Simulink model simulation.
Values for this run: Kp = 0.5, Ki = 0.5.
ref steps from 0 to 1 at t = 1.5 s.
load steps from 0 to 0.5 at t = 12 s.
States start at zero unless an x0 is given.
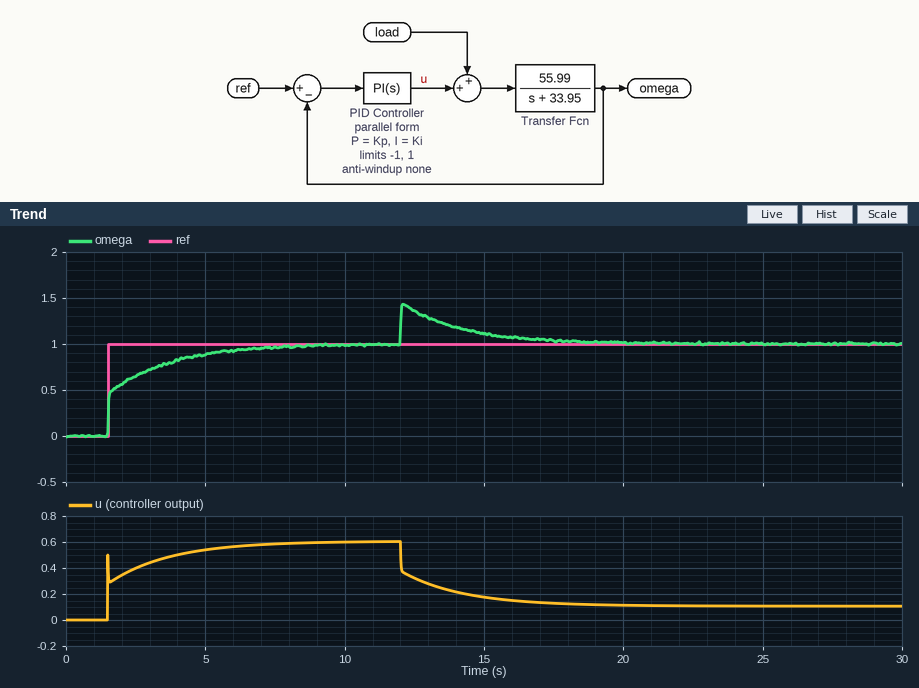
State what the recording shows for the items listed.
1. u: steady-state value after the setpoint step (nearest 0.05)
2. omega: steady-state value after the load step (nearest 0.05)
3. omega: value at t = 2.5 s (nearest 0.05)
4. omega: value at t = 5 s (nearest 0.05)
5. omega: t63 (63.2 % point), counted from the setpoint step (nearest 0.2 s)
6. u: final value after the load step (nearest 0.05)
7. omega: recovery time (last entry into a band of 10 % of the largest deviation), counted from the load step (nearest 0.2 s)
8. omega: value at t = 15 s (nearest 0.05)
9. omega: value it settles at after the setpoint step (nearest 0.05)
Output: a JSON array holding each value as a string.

["0.60", "1.00", "0.65", "0.90", "0.8 s", "0.10", "5.2 s", "1.10", "1.00"]
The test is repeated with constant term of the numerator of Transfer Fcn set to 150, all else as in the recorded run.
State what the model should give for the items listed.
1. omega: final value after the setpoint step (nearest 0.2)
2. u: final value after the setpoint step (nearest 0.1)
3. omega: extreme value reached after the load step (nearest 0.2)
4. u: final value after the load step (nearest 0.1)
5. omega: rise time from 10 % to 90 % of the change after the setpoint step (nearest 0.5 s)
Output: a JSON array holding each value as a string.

["1.0", "0.2", "1.6", "-0.3", "1.5 s"]
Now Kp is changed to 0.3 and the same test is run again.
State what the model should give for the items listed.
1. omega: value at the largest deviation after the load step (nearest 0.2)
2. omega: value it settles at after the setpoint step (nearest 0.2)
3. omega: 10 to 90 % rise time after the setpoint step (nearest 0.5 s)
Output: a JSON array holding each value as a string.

["1.6", "1.0", "3.5 s"]
